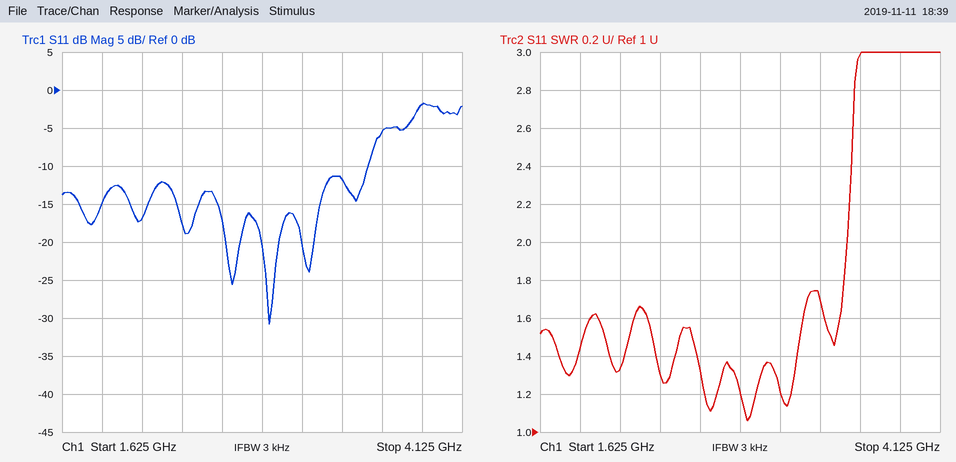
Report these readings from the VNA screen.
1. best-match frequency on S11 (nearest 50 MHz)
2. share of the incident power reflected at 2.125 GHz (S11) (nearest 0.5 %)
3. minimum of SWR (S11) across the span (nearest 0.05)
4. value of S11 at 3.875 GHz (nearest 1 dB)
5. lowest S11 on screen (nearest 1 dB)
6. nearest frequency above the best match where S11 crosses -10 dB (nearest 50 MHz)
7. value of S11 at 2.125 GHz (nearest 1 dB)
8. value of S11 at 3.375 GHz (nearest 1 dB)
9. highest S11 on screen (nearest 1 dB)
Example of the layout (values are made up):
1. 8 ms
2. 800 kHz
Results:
1. 2.90 GHz
2. 2.0 %
3. 1.05
4. -2 dB
5. -31 dB
6. 3.55 GHz
7. -17 dB
8. -12 dB
9. -2 dB
